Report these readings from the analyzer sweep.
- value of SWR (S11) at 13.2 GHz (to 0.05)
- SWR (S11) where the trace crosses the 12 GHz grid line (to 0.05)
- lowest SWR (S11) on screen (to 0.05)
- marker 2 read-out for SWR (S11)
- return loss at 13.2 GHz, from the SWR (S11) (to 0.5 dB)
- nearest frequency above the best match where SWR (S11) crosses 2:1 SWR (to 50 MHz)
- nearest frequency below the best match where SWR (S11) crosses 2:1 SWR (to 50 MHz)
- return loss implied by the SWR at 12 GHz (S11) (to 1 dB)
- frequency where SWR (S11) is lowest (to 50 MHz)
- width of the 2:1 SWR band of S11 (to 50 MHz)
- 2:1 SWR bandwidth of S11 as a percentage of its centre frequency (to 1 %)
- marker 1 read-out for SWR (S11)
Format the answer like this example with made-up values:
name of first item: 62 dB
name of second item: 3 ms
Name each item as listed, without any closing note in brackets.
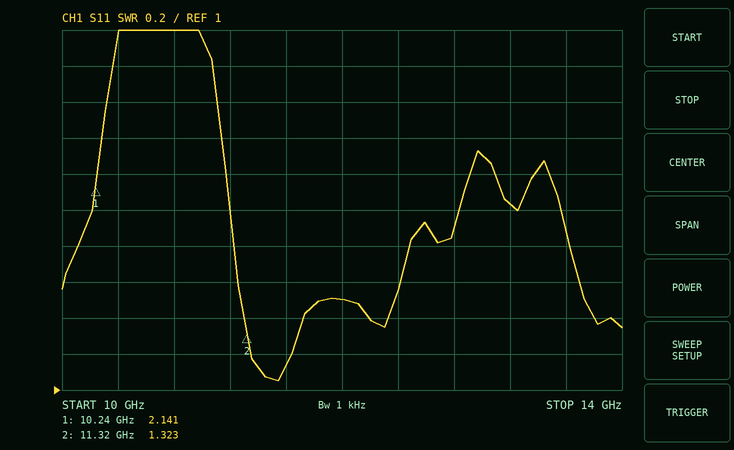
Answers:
value of SWR (S11) at 13.2 GHz: 2.05
SWR (S11) where the trace crosses the 12 GHz grid line: 1.50
lowest SWR (S11) on screen: 1.05
marker 2 read-out for SWR: 1.323
return loss at 13.2 GHz, from the SWR (S11): 9.5 dB
nearest frequency above the best match where SWR (S11) crosses 2:1 SWR: 12.85 GHz
nearest frequency below the best match where SWR (S11) crosses 2:1 SWR: 11.20 GHz
return loss implied by the SWR at 12 GHz (S11): 14 dB
frequency where SWR (S11) is lowest: 11.55 GHz
width of the 2:1 SWR band of S11: 1.65 GHz
2:1 SWR bandwidth of S11 as a percentage of its centre frequency: 14 %
marker 1 read-out for SWR: 2.141
